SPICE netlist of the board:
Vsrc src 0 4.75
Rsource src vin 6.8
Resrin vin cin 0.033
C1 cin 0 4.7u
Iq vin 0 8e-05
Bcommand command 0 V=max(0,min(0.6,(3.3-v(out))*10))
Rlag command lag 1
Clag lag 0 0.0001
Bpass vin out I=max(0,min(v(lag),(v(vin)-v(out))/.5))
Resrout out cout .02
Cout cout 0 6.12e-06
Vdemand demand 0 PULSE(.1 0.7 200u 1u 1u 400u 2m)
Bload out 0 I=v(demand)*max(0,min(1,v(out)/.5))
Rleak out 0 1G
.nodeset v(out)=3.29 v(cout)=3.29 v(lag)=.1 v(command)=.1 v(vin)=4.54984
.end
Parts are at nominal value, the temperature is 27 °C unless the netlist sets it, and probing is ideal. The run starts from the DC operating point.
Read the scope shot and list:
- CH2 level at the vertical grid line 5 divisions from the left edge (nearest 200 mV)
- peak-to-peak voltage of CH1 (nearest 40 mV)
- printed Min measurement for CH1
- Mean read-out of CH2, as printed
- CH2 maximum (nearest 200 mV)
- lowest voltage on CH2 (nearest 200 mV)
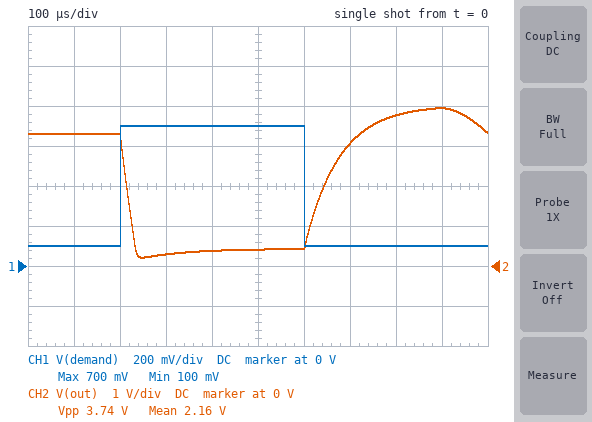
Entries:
400 mV
600 mV
100 mV
2.16 V
4.0 V
200 mV
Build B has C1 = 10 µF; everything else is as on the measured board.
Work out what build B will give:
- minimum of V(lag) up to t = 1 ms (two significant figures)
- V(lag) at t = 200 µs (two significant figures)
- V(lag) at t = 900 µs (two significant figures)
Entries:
60 mV
100 mV
160 mV
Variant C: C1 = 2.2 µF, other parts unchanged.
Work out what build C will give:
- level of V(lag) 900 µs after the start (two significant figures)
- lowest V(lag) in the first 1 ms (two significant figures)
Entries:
76 mV
34 mV
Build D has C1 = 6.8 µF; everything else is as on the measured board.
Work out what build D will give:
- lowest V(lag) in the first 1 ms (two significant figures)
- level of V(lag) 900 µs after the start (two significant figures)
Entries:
44 mV
120 mV
